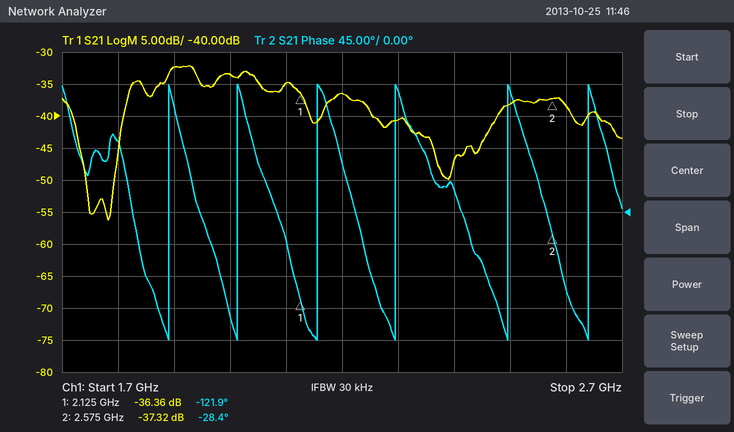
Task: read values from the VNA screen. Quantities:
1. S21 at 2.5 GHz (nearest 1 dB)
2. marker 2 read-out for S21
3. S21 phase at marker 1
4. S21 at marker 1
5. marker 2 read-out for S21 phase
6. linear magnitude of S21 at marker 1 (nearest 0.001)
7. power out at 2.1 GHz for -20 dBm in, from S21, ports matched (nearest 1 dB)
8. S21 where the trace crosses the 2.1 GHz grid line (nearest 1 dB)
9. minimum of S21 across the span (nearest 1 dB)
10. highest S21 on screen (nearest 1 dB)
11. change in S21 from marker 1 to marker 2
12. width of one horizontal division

-38 dB
-37.32 dB
-121.9°
-36.36 dB
-28.4°
0.015
-55 dBm
-35 dB
-56 dB
-32 dB
-0.96 dB
100 MHz
